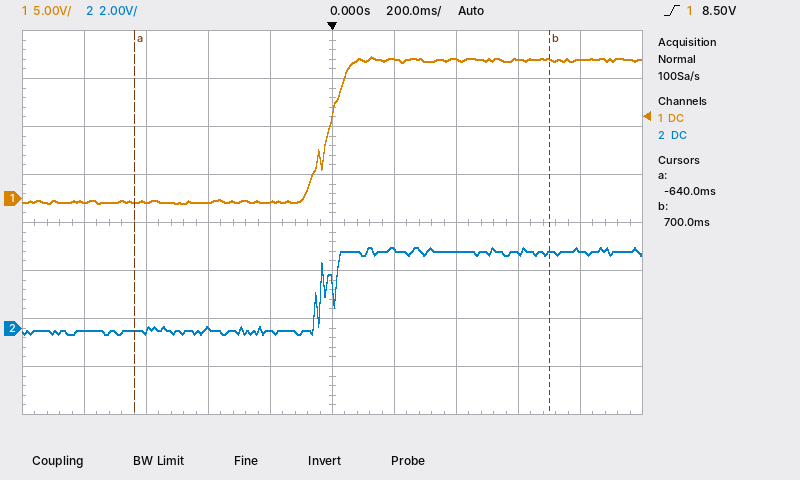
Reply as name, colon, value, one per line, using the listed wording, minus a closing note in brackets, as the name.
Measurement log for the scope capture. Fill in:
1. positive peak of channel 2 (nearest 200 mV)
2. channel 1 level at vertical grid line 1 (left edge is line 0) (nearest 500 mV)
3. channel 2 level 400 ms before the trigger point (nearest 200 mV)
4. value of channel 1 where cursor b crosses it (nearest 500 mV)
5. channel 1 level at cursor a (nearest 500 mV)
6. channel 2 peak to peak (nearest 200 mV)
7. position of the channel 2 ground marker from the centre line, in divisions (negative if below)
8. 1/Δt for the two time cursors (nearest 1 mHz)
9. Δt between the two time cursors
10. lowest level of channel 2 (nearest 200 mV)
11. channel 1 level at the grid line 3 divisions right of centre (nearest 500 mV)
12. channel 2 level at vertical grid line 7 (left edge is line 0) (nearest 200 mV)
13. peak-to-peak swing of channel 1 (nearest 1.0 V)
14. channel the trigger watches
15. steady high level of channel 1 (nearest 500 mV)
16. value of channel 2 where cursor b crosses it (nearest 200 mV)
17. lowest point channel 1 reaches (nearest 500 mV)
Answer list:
positive peak of channel 2: 3.4 V
channel 1 level at vertical grid line 1 (left edge is line 0): -500 mV
channel 2 level 400 ms before the trigger point: 0.0 V
value of channel 1 where cursor b crosses it: 14.5 V
channel 1 level at cursor a: -500 mV
channel 2 peak to peak: 3.6 V
position of the channel 2 ground marker from the centre line, in divisions: -2.2 div
1/Δt for the two time cursors: 746 mHz
Δt between the two time cursors: 1.34 s
lowest level of channel 2: -200 mV
channel 1 level at the grid line 3 divisions right of centre: 14.5 V
channel 2 level at vertical grid line 7 (left edge is line 0): 3.2 V
peak-to-peak swing of channel 1: 15.0 V
channel the trigger watches: channel 1
steady high level of channel 1: 14.5 V
value of channel 2 where cursor b crosses it: 3.2 V
lowest point channel 1 reaches: -500 mV
